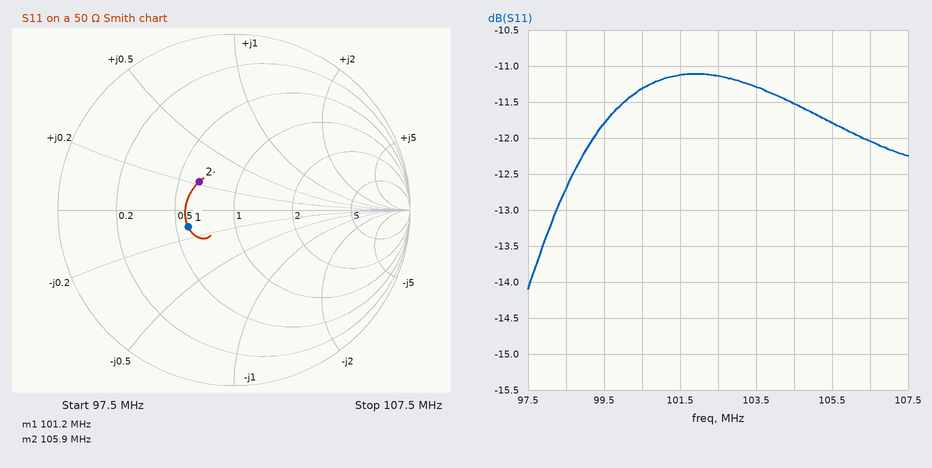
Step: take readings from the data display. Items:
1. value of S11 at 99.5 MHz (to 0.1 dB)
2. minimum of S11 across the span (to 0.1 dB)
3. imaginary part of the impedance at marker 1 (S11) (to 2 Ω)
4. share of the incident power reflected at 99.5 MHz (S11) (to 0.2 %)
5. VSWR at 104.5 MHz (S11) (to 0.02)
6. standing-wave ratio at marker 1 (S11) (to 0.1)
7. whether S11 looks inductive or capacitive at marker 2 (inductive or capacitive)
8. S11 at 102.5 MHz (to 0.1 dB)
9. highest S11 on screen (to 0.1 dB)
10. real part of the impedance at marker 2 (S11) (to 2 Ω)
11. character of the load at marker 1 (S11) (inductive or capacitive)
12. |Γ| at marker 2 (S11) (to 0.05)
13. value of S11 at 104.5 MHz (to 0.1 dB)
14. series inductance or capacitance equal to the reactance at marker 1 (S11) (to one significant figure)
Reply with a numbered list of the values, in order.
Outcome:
1. -11.8 dB
2. -14.1 dB
3. -6 Ω
4. 6.6 %
5. 1.72
6. 1.8
7. inductive
8. -11.1 dB
9. -11.1 dB
10. 32 Ω
11. capacitive
12. 0.25
13. -11.5 dB
14. 300 pF
